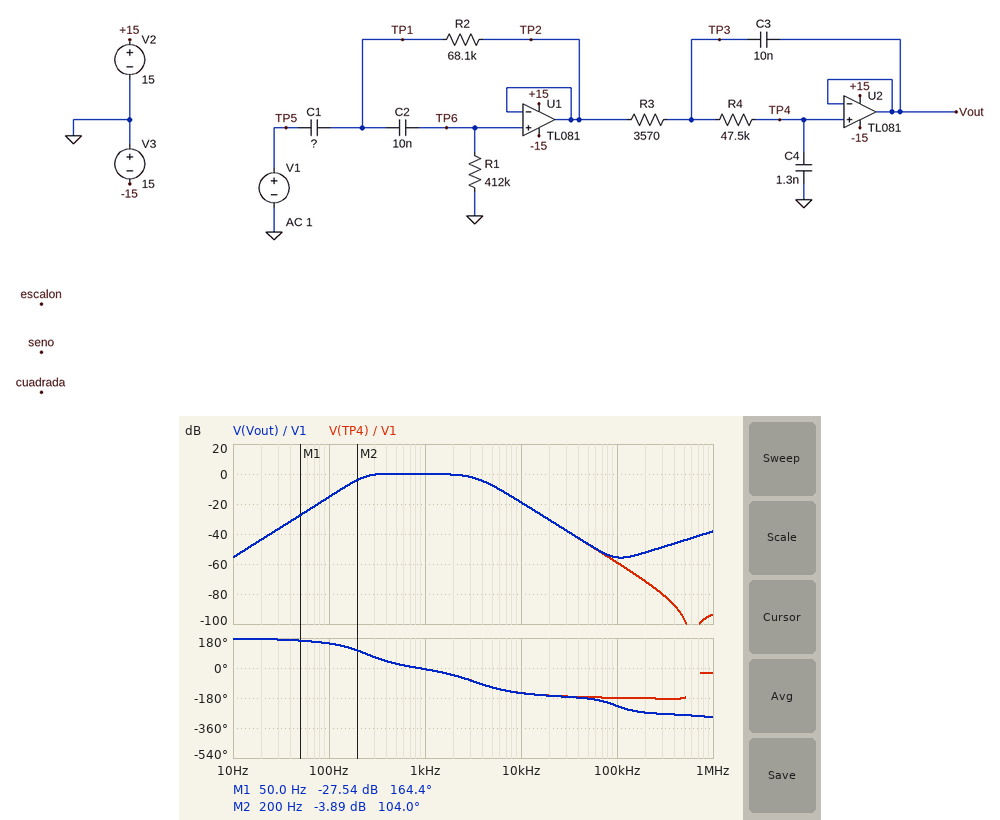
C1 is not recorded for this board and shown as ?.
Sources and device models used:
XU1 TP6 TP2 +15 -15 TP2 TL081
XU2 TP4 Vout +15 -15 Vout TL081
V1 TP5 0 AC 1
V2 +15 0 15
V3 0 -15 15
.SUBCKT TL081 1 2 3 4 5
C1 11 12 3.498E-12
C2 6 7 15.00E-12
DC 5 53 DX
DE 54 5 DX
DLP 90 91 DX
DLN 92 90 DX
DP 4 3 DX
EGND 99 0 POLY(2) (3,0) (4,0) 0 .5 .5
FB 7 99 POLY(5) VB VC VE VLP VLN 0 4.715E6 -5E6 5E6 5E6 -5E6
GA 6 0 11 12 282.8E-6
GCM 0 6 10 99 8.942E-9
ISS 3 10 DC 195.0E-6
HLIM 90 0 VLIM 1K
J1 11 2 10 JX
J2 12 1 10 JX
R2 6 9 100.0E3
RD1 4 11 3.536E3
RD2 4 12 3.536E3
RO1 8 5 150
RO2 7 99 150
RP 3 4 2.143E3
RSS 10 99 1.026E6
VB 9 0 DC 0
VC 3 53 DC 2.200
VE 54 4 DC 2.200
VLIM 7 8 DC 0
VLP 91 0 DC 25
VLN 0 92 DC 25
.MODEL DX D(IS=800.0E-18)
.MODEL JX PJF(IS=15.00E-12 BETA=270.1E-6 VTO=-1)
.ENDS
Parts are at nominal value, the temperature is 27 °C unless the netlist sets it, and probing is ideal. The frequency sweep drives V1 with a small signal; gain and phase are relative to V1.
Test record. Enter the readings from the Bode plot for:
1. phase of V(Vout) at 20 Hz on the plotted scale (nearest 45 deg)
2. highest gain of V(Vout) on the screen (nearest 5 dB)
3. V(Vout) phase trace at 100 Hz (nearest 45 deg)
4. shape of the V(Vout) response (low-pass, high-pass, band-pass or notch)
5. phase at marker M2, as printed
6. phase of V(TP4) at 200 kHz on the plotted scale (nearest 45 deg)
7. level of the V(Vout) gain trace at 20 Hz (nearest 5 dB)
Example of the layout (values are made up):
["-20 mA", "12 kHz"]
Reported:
["180 deg", "0 dB", "135 deg", "band-pass", "104.0 deg", "-180 deg", "-45 dB"]
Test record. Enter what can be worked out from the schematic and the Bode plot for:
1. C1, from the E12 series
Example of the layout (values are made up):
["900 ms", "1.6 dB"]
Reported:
["1.5 nF"]
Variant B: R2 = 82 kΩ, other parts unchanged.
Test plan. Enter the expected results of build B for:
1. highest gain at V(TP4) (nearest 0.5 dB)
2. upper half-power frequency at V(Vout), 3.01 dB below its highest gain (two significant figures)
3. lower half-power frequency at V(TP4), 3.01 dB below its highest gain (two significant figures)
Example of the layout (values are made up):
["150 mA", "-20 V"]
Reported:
["0 dB", "3.4 kHz", "210 Hz"]
